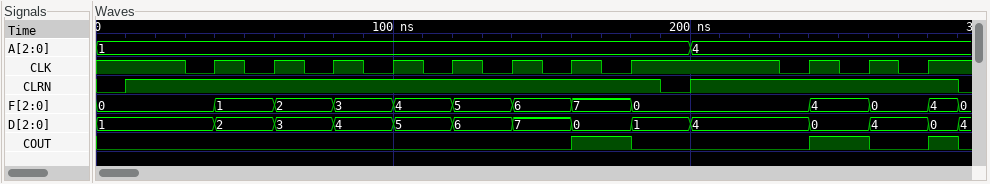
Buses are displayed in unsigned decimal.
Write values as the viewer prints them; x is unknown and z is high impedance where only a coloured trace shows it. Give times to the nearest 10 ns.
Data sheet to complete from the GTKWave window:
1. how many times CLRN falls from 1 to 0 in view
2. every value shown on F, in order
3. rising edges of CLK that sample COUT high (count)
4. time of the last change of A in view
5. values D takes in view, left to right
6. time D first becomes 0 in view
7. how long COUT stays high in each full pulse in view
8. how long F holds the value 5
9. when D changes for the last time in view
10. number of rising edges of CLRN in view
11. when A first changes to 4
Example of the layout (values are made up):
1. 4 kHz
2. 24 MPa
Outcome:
1. 2
2. 0, 1, 2, 3, 4, 5, 6, 7, 0, 4, 0, 4, 0
3. 2
4. 200 ns
5. 1, 2, 3, 4, 5, 6, 7, 0, 1, 4, 0, 4, 0, 4
6. 160 ns
7. 20 ns, 20 ns, 10 ns
8. 20 ns
9. 290 ns
10. 2
11. 200 ns
